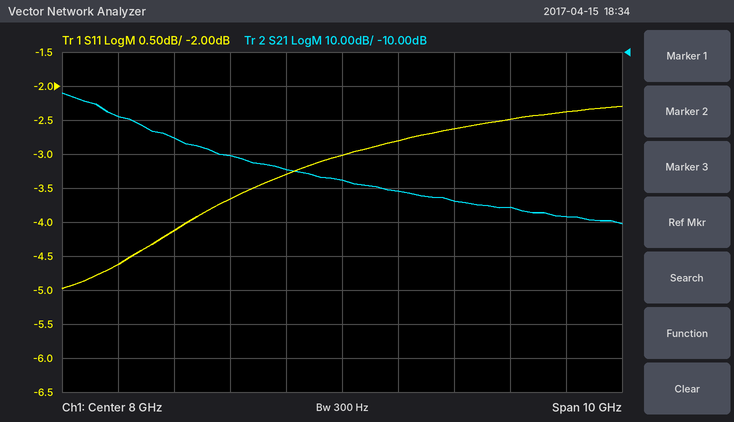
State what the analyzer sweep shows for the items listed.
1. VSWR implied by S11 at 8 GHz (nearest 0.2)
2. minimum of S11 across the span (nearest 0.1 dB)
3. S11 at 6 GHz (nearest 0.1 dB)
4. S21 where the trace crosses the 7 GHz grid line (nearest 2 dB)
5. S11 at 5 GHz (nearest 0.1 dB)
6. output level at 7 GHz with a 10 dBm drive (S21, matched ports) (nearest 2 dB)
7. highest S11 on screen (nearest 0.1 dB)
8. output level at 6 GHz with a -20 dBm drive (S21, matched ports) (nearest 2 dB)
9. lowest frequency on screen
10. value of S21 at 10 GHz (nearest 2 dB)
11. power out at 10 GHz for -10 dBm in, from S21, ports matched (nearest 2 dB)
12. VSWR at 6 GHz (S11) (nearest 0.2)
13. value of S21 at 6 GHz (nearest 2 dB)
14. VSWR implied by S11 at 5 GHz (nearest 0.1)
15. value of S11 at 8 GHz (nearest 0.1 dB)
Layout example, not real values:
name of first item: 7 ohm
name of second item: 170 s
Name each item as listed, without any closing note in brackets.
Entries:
VSWR implied by S11 at 8 GHz: 5.8
minimum of S11 across the span: -5.0 dB
S11 at 6 GHz: -3.7 dB
S21 where the trace crosses the 7 GHz grid line: -44 dB
S11 at 5 GHz: -4.1 dB
output level at 7 GHz with a 10 dBm drive (S21, matched ports): -34 dBm
highest S11 on screen: -2.3 dB
output level at 6 GHz with a -20 dBm drive (S21, matched ports): -60 dBm
lowest frequency on screen: 3 GHz
value of S21 at 10 GHz: -54 dB
power out at 10 GHz for -10 dBm in, from S21, ports matched: -64 dBm
VSWR at 6 GHz (S11): 4.8
value of S21 at 6 GHz: -40 dB
VSWR implied by S11 at 5 GHz: 4.3
value of S11 at 8 GHz: -3.0 dB
